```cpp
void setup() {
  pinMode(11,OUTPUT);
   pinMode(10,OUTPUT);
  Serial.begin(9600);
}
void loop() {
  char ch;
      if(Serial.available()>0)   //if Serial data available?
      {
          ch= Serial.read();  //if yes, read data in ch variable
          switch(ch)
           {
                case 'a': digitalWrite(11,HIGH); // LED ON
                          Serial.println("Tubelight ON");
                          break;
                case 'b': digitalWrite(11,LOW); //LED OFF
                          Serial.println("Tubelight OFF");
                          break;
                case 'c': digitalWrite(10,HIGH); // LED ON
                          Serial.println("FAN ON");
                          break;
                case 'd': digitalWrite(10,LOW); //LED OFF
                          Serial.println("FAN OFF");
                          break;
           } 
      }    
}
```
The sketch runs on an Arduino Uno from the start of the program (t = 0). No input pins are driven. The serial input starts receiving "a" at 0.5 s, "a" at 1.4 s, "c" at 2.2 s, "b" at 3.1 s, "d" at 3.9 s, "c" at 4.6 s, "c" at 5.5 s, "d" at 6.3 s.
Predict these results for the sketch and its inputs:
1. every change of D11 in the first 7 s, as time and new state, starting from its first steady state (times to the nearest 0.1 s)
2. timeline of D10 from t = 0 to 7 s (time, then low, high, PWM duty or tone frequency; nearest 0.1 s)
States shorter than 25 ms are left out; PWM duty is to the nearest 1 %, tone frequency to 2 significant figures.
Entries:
0 s low; 0.5 s high; 3.1 s low
0 s low; 2.2 s high; 3.9 s low; 4.6 s high; 6.3 s low
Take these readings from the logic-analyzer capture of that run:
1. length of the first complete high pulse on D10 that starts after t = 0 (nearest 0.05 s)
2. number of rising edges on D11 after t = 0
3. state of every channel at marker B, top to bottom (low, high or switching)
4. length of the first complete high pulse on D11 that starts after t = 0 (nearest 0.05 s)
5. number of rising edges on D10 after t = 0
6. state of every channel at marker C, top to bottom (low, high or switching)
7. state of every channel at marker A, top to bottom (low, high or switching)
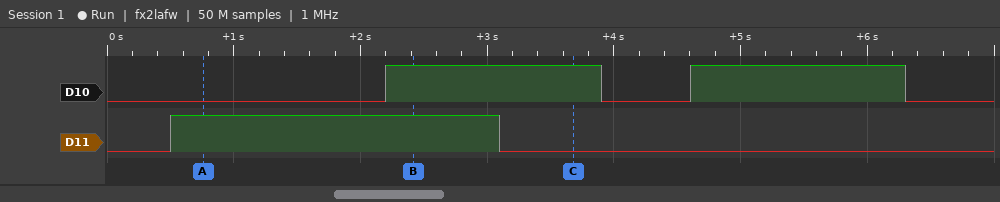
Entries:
1.70 s
1
D10 high, D11 high
2.60 s
2
D10 high, D11 low
D10 low, D11 high
